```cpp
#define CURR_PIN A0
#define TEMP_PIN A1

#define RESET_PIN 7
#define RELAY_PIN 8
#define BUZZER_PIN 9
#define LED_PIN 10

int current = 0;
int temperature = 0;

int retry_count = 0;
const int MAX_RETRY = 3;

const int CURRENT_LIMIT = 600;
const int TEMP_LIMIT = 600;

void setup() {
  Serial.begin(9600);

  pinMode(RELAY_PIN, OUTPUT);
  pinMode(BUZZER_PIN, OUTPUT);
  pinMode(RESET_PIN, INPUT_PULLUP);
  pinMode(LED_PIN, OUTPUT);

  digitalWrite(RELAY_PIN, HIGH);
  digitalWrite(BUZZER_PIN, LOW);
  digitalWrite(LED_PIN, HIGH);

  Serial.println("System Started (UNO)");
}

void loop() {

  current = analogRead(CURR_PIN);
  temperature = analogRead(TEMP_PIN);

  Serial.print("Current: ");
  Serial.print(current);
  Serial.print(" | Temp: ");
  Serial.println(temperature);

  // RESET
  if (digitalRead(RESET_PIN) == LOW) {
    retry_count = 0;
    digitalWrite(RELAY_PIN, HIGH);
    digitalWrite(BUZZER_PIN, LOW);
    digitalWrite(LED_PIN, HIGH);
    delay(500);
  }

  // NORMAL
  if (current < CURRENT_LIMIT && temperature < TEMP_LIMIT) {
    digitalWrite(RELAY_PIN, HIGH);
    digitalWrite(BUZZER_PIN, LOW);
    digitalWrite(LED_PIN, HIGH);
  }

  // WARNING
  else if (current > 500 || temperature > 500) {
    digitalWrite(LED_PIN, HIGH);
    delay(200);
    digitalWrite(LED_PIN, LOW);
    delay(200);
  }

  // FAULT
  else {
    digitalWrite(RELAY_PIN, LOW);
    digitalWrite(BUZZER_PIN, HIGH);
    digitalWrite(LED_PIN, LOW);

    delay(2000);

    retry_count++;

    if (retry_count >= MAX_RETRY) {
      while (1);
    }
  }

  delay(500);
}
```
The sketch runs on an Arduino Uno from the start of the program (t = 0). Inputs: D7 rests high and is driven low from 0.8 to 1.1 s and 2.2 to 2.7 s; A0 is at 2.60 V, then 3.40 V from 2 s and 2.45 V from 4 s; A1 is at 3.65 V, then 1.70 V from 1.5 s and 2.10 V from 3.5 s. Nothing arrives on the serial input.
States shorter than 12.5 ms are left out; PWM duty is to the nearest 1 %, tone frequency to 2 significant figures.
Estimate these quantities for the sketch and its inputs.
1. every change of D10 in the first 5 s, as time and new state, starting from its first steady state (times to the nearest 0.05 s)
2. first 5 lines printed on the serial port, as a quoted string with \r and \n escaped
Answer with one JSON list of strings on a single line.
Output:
["0 s high; 0.2 s low; 0.9 s high; 1.6 s low; 2.3 s high; 3 s low; 3.7 s high; 3.9 s low; 4.6 s high", "\"System Started (UNO)\\r\\nCurrent: 532 | Temp: 747\\r\\nCurrent: 532 | Temp: 747\\r\\nCurrent: 696 | Temp: 348\\r\\nCurrent: 696 | Temp: 430\\r\\n\""]
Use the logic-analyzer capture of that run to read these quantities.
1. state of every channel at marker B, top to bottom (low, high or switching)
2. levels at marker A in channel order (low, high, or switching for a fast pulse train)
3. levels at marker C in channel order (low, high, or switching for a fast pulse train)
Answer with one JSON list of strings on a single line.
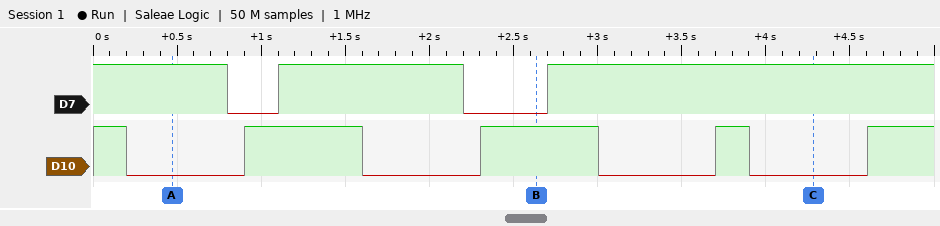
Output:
["D7 low, D10 high", "D7 high, D10 low", "D7 high, D10 low"]
